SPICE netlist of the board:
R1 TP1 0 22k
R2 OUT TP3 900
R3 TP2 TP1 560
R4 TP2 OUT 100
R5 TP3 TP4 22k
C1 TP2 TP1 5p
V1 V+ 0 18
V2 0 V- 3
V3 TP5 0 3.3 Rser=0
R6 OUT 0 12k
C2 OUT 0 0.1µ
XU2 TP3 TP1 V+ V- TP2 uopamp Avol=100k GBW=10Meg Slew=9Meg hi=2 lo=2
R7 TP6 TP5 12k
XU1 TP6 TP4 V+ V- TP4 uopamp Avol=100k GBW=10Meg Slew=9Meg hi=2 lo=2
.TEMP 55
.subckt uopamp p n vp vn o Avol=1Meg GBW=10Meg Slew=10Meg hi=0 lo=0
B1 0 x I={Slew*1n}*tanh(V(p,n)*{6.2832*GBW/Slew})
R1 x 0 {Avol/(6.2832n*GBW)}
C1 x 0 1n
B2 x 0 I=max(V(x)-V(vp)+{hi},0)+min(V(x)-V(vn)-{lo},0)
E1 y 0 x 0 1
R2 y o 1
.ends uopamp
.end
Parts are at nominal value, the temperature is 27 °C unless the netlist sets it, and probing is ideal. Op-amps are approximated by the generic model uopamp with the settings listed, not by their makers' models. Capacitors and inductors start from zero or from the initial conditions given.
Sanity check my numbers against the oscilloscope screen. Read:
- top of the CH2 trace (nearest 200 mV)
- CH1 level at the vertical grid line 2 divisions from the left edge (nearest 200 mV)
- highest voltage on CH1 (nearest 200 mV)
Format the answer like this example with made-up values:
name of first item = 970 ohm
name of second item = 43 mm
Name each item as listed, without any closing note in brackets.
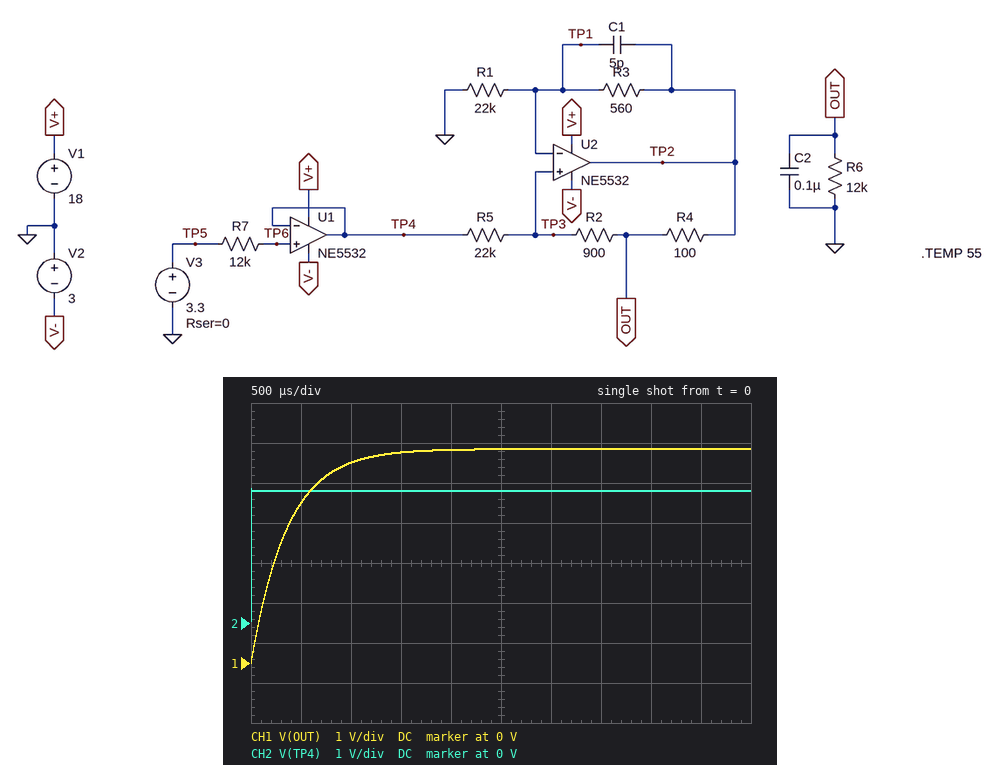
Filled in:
top of the CH2 trace = 3.4 V
CH1 level at the vertical grid line 2 divisions from the left edge = 5.0 V
highest voltage on CH1 = 5.4 V
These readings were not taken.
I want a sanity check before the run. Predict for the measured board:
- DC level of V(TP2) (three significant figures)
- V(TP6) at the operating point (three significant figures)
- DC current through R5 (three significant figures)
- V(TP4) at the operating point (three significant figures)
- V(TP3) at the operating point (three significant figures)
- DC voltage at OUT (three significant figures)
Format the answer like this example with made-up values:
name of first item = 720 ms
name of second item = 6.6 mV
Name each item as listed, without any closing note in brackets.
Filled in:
DC level of V(TP2) = 5.40 V
V(TP6) at the operating point = 3.30 V
DC current through R5 = 89.5 µA
V(TP4) at the operating point = 3.30 V
V(TP3) at the operating point = 5.27 V
DC voltage at OUT = 5.35 V
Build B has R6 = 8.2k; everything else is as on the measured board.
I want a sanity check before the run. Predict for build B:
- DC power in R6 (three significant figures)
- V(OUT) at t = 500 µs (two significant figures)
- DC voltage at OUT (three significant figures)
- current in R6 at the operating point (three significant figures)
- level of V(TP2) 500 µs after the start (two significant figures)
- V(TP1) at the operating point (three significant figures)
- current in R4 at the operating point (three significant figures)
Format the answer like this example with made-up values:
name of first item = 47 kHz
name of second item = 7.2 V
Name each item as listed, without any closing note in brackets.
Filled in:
DC power in R6 = 2.68 mW
V(OUT) at t = 500 µs = 3.7 V
DC voltage at OUT = 4.69 V
current in R6 at the operating point = 572 µA
level of V(TP2) 500 µs after the start = 3.8 V
V(TP1) at the operating point = 4.64 V
current in R4 at the operating point = 633 µA
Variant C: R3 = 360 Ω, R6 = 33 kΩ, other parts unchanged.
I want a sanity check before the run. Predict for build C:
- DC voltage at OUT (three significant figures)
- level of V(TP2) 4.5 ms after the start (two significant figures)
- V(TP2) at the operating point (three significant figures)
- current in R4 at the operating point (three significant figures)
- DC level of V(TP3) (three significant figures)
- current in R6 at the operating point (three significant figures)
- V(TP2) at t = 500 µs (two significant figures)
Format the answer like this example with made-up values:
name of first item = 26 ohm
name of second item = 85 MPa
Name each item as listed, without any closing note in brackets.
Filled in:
DC voltage at OUT = 4.72 V
level of V(TP2) 4.5 ms after the start = 4.7 V
V(TP2) at the operating point = 4.74 V
current in R4 at the operating point = 205 µA
DC level of V(TP3) = 4.66 V
current in R6 at the operating point = 143 µA
V(TP2) at t = 500 µs = 3.8 V
